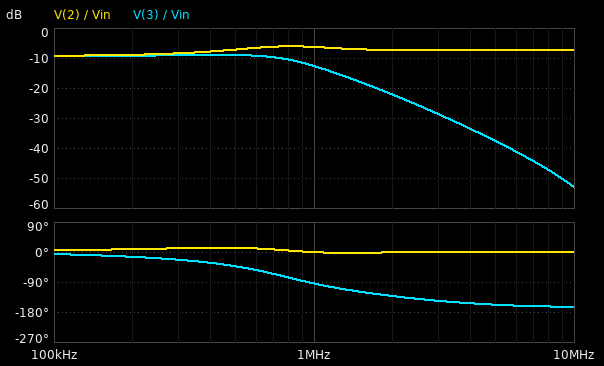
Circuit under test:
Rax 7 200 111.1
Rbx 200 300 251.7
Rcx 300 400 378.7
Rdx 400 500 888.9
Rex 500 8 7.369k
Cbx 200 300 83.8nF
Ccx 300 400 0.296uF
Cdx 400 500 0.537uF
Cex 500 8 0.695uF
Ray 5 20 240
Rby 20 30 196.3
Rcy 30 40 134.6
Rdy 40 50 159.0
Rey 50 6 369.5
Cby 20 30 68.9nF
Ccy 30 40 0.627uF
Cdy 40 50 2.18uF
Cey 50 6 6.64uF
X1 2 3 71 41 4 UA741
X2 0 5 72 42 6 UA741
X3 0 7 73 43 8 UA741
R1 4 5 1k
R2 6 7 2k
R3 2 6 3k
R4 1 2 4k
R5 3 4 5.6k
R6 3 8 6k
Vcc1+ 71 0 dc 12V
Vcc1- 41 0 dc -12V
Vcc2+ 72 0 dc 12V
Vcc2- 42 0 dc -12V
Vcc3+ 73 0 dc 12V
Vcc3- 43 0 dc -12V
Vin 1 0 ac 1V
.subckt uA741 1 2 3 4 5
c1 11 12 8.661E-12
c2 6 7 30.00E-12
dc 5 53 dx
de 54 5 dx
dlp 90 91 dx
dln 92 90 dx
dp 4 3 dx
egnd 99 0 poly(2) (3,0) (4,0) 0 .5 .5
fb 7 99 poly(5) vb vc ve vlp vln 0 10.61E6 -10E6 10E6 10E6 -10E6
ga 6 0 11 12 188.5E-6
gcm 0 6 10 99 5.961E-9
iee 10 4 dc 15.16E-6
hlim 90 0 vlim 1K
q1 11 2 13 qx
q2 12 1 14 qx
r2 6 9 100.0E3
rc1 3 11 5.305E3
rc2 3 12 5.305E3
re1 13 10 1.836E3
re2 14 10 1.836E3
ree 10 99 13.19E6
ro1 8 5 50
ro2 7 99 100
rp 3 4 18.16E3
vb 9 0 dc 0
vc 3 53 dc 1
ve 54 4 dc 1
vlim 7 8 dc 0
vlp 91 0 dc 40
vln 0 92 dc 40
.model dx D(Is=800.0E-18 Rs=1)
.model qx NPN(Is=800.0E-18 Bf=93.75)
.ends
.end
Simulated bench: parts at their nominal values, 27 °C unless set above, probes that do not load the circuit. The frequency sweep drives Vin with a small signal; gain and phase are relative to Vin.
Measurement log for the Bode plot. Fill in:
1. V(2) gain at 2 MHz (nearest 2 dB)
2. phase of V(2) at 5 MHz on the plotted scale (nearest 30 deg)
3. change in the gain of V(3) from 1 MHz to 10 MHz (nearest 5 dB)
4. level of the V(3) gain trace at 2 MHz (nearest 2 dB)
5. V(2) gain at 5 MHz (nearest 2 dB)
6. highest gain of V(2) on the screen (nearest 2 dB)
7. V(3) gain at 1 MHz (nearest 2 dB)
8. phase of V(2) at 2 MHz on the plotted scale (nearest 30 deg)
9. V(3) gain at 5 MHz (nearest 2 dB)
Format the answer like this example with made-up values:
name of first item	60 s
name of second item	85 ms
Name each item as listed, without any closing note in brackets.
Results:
V(2) gain at 2 MHz	-8 dB
phase of V(2) at 5 MHz on the plotted scale	0 deg
change in the gain of V(3) from 1 MHz to 10 MHz	-40 dB
level of the V(3) gain trace at 2 MHz	-22 dB
V(2) gain at 5 MHz	-8 dB
highest gain of V(2) on the screen	-6 dB
V(3) gain at 1 MHz	-12 dB
phase of V(2) at 2 MHz on the plotted scale	0 deg
V(3) gain at 5 MHz	-38 dB
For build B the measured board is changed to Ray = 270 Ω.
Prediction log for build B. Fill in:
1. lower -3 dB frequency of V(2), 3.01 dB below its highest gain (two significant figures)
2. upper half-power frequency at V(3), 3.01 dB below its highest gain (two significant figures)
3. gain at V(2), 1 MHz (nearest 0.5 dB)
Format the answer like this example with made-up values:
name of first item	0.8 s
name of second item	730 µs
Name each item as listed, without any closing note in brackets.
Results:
lower -3 dB frequency of V(2), 3.01 dB below its highest gain	230 kHz
upper half-power frequency at V(3), 3.01 dB below its highest gain	950 kHz
gain at V(2), 1 MHz	-6.0 dB
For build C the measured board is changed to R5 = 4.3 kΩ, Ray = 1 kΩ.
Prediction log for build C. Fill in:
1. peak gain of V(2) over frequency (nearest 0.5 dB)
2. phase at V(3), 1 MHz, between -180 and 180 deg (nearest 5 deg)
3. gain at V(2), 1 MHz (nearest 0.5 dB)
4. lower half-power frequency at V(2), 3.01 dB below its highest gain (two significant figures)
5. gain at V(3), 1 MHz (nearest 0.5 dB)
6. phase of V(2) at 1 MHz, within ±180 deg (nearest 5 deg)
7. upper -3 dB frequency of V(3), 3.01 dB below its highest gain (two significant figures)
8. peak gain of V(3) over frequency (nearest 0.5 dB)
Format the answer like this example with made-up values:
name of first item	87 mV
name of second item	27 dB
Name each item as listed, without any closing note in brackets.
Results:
peak gain of V(2) over frequency	-3.5 dB
phase at V(3), 1 MHz, between -180 and 180 deg	-95 deg
gain at V(2), 1 MHz	-4.5 dB
lower half-power frequency at V(2), 3.01 dB below its highest gain	550 kHz
gain at V(3), 1 MHz	-10.0 dB
phase of V(2) at 1 MHz, within ±180 deg	-5 deg
upper -3 dB frequency of V(3), 3.01 dB below its highest gain	970 kHz
peak gain of V(3) over frequency	-6.5 dB
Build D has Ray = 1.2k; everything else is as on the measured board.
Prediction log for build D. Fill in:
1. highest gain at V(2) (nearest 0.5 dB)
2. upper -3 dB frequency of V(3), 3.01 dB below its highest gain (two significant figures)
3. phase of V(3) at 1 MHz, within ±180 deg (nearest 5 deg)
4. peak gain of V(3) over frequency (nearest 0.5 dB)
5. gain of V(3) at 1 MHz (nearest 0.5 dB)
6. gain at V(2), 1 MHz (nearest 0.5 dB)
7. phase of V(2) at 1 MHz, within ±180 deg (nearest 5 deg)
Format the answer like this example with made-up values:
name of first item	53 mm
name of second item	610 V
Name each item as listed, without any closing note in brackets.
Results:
highest gain at V(2)	-2.0 dB
upper -3 dB frequency of V(3), 3.01 dB below its highest gain	900 kHz
phase of V(3) at 1 MHz, within ±180 deg	-100 deg
peak gain of V(3) over frequency	-6.0 dB
gain of V(3) at 1 MHz	-11.0 dB
gain at V(2), 1 MHz	-4.5 dB
phase of V(2) at 1 MHz, within ±180 deg	-5 deg
